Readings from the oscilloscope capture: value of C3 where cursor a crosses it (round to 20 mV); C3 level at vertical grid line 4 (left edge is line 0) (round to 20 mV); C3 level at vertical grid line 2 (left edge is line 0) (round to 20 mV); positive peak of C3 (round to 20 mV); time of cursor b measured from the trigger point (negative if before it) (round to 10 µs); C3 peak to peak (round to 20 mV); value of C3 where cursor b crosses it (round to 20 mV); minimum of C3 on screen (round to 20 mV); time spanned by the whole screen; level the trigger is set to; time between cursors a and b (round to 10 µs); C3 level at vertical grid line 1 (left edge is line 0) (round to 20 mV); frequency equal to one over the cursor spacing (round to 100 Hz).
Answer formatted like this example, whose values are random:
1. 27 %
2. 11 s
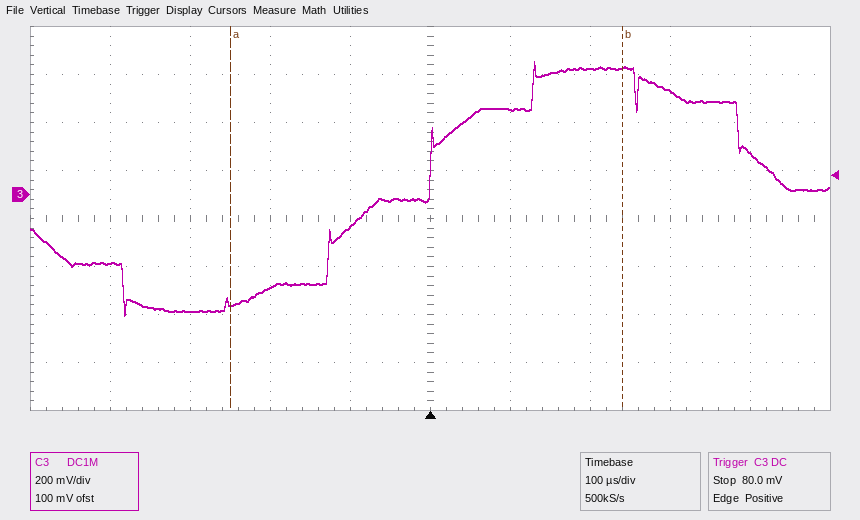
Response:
1. -440 mV
2. -140 mV
3. -480 mV
4. 560 mV
5. +240 µs
6. 1.06 V
7. 520 mV
8. -500 mV
9. 1 ms
10. 80.0 mV
11. 490 µs
12. -280 mV
13. 2.0 kHz
